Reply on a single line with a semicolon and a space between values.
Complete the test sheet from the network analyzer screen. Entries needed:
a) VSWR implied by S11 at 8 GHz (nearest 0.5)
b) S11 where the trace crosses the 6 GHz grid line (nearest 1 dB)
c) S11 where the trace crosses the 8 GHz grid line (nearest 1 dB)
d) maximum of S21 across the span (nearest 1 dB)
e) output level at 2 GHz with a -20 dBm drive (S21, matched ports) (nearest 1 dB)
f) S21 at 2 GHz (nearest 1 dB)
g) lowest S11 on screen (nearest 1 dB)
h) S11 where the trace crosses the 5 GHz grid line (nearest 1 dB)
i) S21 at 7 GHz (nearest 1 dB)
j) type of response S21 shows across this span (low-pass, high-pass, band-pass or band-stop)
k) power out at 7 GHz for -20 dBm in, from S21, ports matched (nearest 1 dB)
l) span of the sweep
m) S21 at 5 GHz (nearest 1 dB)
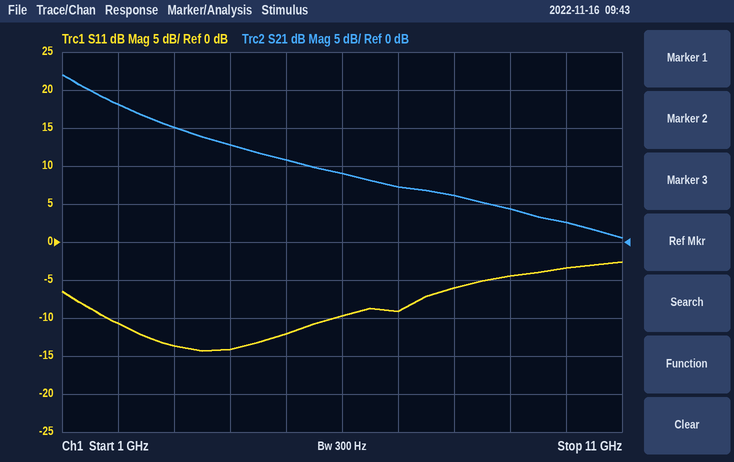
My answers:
3.0; -10 dB; -6 dB; 22 dB; -2 dBm; 18 dB; -14 dB; -12 dB; 7 dB; low-pass; -13 dBm; 10 GHz; 11 dB
